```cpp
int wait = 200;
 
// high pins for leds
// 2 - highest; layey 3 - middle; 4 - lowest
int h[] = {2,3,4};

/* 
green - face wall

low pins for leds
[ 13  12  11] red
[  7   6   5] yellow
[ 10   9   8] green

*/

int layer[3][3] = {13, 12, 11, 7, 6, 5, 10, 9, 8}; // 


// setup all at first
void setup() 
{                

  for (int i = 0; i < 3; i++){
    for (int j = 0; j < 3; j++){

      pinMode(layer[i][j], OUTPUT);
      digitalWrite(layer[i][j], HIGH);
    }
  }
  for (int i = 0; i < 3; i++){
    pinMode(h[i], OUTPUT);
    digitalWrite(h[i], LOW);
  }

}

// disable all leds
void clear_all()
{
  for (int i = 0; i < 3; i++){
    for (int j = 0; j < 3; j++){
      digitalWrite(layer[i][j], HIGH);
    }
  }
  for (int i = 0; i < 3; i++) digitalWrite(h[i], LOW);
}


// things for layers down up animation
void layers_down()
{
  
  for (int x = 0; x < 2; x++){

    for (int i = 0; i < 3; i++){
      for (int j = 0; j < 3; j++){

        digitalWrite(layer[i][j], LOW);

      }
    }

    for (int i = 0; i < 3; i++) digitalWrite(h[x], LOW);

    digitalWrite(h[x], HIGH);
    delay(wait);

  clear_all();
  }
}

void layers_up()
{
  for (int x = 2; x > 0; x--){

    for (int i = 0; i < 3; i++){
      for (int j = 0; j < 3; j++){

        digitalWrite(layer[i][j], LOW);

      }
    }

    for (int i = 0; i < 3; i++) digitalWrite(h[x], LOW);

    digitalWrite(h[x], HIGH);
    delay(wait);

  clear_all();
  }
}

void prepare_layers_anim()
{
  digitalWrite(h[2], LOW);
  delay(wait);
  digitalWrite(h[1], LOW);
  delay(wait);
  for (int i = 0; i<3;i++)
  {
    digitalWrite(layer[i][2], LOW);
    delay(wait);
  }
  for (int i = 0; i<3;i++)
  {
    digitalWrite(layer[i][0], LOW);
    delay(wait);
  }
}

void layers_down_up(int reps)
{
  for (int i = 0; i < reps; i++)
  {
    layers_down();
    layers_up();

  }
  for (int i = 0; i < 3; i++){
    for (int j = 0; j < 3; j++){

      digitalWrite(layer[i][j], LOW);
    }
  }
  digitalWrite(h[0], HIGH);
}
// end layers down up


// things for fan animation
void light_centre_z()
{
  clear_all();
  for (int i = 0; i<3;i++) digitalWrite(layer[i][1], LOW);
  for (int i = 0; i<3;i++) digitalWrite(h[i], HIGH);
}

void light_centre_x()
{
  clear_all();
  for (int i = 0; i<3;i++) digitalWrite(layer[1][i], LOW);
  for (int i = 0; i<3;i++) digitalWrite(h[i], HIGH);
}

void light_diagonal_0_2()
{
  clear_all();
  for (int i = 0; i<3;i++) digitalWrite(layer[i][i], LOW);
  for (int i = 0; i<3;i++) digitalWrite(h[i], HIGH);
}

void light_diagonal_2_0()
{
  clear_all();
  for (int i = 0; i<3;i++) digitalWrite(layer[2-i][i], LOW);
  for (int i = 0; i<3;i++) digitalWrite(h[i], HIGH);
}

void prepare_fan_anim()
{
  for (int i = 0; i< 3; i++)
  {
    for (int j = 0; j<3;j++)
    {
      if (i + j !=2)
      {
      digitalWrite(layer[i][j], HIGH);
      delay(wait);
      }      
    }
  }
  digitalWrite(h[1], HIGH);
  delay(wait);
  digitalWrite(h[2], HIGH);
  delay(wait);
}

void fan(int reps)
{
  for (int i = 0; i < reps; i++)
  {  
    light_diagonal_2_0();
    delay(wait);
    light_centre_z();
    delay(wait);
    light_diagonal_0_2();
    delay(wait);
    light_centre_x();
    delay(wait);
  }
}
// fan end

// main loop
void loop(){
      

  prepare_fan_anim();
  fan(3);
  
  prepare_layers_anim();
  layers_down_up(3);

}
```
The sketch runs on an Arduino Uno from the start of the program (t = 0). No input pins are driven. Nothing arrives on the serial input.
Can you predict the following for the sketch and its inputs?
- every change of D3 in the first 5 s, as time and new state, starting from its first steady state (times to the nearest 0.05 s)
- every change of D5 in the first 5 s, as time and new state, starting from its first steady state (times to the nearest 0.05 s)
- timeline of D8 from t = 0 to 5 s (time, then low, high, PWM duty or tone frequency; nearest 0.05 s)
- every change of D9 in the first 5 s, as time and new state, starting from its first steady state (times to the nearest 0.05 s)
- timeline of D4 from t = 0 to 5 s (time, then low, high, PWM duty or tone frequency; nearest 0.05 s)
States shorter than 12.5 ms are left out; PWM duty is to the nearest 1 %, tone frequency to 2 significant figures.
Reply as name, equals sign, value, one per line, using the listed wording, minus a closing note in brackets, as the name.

every change of D3 in the first 5 s, as time and new state, starting from its first steady state = 0 s low; 1.2 s high; 4.2 s low
every change of D5 in the first 5 s, as time and new state, starting from its first steady state = 0 s high; 2.2 s low; 2.4 s high; 3 s low; 3.2 s high; 3.8 s low
timeline of D8 from t = 0 to 5 s = 0 s high; 2 s low; 2.2 s high; 2.8 s low; 3 s high; 3.6 s low; 3.8 s high; 4.8 s low
every change of D9 in the first 5 s, as time and new state, starting from its first steady state = 0 s high; 1.8 s low; 2 s high; 2.6 s low; 2.8 s high; 3.4 s low; 3.6 s high
timeline of D4 from t = 0 to 5 s = 0 s low; 1.4 s high; 4 s low
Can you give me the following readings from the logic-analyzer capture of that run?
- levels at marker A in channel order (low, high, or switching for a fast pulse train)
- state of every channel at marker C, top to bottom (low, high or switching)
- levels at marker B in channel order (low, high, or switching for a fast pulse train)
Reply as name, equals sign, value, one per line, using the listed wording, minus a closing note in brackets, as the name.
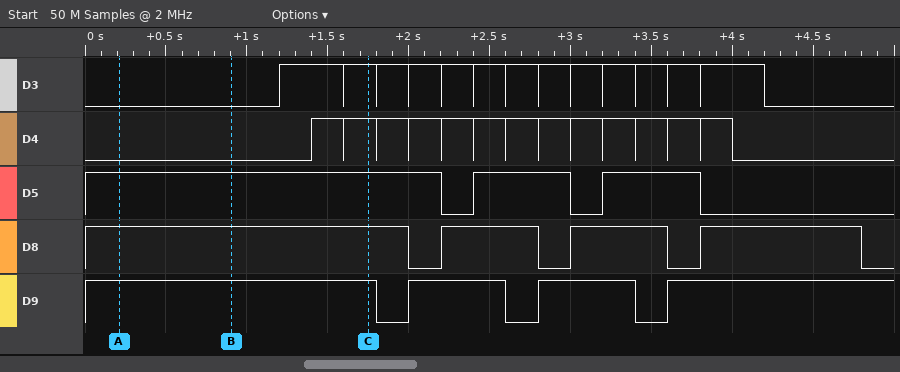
levels at marker A in channel order = D3 low, D4 low, D5 high, D8 high, D9 high
state of every channel at marker C, top to bottom = D3 high, D4 high, D5 high, D8 high, D9 high
levels at marker B in channel order = D3 low, D4 low, D5 high, D8 high, D9 high
